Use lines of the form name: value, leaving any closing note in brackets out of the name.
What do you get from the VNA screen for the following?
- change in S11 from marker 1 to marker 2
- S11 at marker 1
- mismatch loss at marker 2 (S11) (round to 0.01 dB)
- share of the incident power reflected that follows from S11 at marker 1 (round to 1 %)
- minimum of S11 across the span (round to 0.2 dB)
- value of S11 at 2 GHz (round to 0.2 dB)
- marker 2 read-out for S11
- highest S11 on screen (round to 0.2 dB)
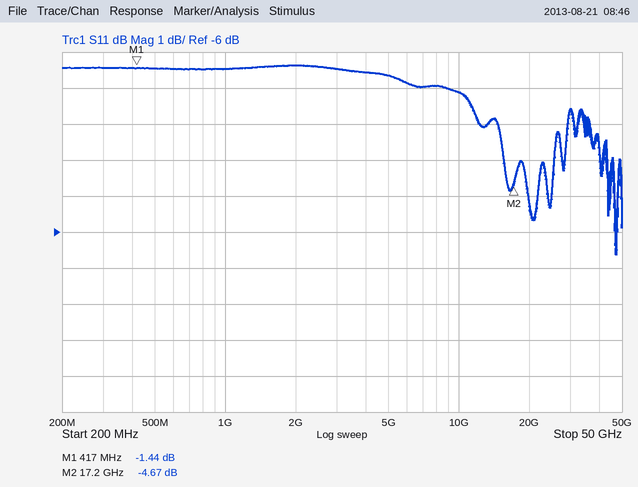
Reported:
change in S11 from marker 1 to marker 2: -3.23 dB
S11 at marker 1: -1.44 dB
mismatch loss at marker 2 (S11): 1.81 dB
share of the incident power reflected that follows from S11 at marker 1: 72 %
minimum of S11 across the span: -6.6 dB
value of S11 at 2 GHz: -1.4 dB
marker 2 read-out for S11: -4.67 dB
highest S11 on screen: -1.4 dB
